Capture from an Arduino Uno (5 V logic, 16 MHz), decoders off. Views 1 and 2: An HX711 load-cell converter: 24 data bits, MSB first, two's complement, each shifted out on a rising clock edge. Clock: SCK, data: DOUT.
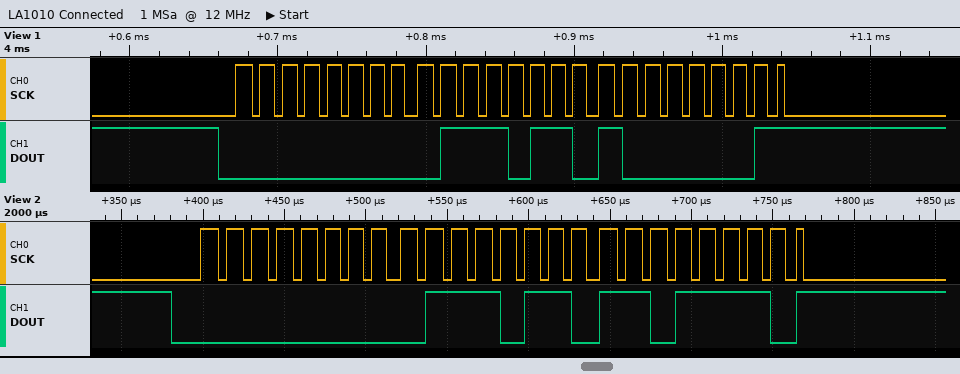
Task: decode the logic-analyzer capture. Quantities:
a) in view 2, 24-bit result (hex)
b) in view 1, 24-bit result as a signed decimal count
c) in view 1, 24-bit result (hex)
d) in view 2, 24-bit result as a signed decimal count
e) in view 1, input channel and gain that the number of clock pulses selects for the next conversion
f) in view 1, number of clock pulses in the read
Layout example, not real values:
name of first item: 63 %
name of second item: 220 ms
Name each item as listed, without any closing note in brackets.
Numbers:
in view 2, 24-bit result: 0x0076DE
in view 1, 24-bit result as a signed decimal count: 30337
in view 1, 24-bit result: 0x007681
in view 2, 24-bit result as a signed decimal count: 30430
in view 1, input channel and gain that the number of clock pulses selects for the next conversion: channel A, gain 128
in view 1, number of clock pulses in the read: 25
